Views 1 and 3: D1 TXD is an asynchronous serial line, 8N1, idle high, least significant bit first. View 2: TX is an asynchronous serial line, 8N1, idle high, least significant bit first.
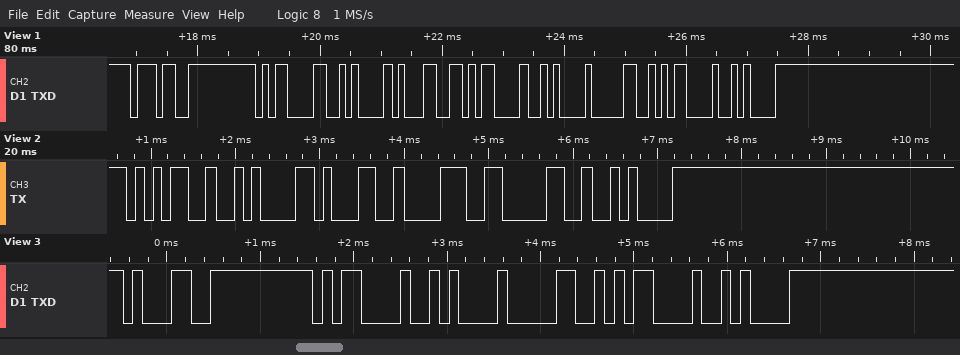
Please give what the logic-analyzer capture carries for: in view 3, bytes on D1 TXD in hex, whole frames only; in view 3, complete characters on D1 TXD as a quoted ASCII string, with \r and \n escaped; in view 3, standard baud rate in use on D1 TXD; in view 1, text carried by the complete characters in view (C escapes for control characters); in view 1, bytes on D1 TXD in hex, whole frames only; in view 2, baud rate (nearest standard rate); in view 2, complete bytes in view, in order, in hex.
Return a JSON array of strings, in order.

["31 0D 0A 30 0D 0A", "\"1\\r\\n0\\r\\n\"", "9600 baud", "\"7\\r\\n1\\r\\n0\\r\\n\"", "37 0D 0A 31 0D 0A 30 0D 0A", "9600 baud", "35 0A 31 38 30 0A"]
